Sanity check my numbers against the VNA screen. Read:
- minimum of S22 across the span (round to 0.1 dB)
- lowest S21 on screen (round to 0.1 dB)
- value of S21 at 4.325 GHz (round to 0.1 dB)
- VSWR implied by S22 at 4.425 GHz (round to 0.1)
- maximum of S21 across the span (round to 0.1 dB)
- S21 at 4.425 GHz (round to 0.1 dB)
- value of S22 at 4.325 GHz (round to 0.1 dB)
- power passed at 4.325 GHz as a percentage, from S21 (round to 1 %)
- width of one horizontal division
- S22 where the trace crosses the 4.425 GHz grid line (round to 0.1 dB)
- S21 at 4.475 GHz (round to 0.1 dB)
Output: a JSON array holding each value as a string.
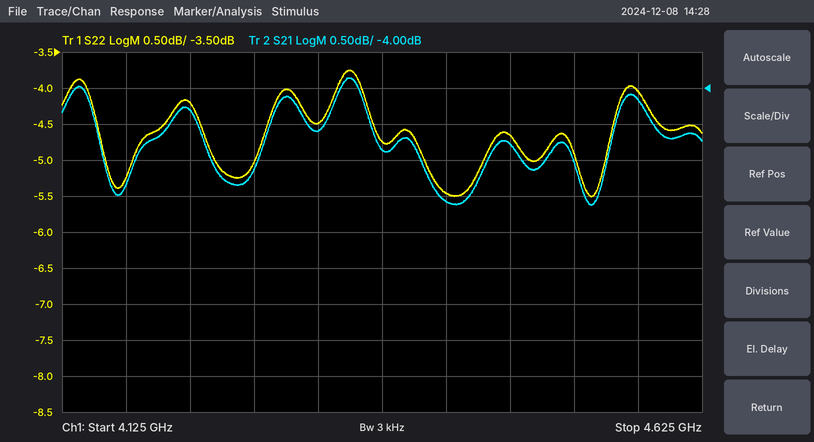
["-5.5 dB", "-5.6 dB", "-4.6 dB", "3.3", "-3.9 dB", "-5.6 dB", "-4.5 dB", "35 %", "50 MHz", "-5.5 dB", "-4.8 dB"]
